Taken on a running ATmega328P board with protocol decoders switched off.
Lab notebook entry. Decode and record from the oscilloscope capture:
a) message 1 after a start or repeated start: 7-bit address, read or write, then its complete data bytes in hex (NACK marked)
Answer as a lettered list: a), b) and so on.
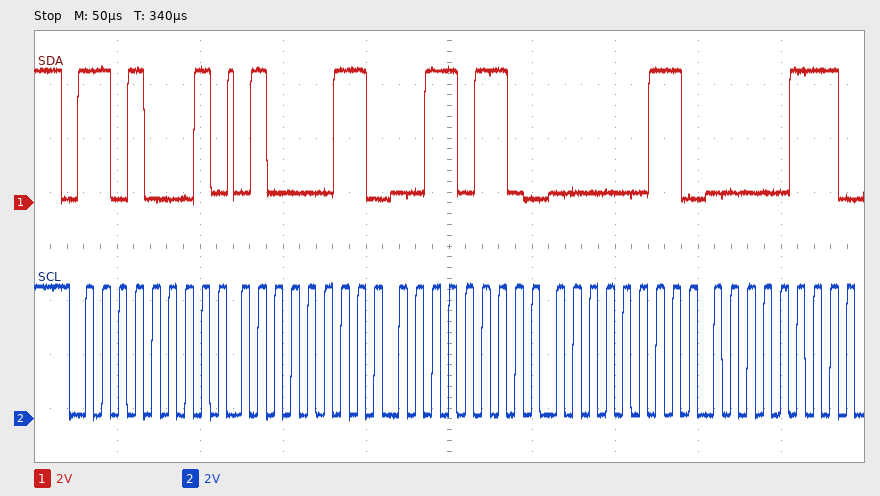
a) 0x68 read: 43 36 03 07
